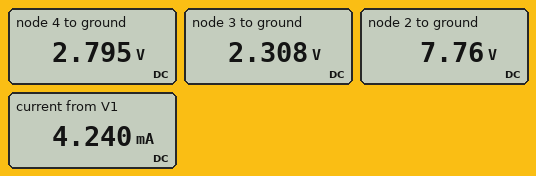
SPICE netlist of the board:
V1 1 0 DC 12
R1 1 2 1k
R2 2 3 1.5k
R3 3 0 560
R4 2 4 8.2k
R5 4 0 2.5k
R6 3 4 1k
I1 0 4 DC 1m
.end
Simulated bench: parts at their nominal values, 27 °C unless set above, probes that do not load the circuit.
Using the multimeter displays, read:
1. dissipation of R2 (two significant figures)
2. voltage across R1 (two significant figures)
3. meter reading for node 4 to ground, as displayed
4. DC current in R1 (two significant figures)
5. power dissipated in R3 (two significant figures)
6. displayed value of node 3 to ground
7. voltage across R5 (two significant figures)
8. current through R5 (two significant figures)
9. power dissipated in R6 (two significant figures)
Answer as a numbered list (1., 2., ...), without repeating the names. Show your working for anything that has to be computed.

1. (7.76 V - 2.308 V)^2 / 1.5 kΩ = 20 mW
2. 12 V - 7.76 V = 4.2 V
3. 2.795 V
4. (12 V - 7.76 V) / 1 kΩ = 4.2 mA
5. (2.308 V)^2 / 560 Ω = 9.5 mW
6. 2.308 V
7. 2.795 V = 2.8 V
8. (2.795 V) / 2.5 kΩ = 1.1 mA
9. (2.795 V - 2.308 V)^2 / 1 kΩ = 240 µW
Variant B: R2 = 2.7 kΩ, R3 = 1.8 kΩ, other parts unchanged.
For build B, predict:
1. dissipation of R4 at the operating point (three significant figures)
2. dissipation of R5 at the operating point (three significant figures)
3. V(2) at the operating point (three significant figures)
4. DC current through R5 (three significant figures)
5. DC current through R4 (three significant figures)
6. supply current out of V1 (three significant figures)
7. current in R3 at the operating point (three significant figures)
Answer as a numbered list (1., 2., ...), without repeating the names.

1. 3.55 mW
2. 6.13 mW
3. 9.31 V
4. 1.57 mA
5. 658 µA
6. 2.69 mA
7. 2.12 mA
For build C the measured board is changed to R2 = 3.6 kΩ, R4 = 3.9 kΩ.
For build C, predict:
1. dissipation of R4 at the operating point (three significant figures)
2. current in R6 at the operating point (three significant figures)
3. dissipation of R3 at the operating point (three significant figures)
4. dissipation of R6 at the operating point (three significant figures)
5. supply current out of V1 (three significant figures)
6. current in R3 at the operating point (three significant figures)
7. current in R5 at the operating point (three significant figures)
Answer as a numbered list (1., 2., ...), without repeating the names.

1. 8.15 mW
2. 1.24 mA
3. 5.57 mW
4. 1.54 mW
5. 3.36 mA
6. 3.15 mA
7. 1.20 mA
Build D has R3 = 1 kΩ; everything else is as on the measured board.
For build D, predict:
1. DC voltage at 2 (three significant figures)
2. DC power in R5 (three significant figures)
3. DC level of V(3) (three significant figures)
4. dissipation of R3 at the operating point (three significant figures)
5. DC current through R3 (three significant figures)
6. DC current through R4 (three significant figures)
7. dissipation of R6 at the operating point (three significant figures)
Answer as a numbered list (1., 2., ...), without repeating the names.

1. 8.21 V
2. 5.00 mW
3. 3.38 V
4. 11.4 mW
5. 3.38 mA
6. 570 µA
7. 24.5 µW
